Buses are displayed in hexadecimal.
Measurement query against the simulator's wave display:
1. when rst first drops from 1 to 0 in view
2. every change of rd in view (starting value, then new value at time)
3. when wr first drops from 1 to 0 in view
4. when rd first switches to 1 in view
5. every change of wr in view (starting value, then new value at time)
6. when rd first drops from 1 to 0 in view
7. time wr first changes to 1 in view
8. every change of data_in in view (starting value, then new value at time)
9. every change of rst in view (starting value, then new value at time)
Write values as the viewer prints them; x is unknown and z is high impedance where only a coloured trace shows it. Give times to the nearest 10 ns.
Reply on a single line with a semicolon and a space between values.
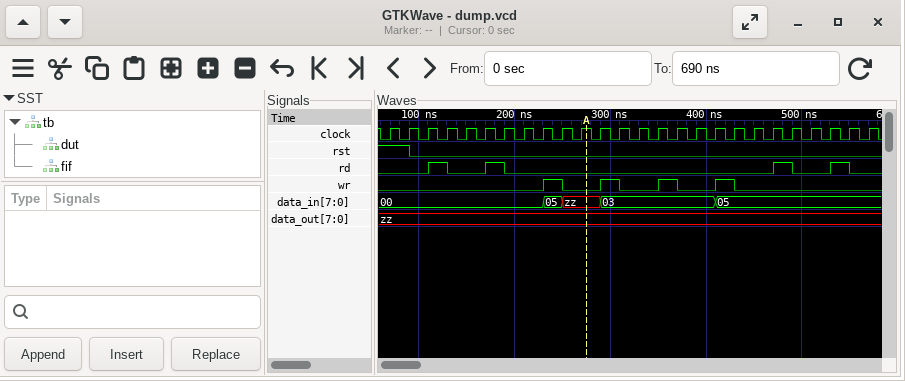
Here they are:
90 ns; 0, 1 at 110 ns, 0 at 130 ns, 1 at 170 ns, 0 at 190 ns, 1 at 470 ns, 0 at 490 ns, 1 at 530 ns, 0 at 550 ns; 250 ns; 110 ns; 0, 1 at 230 ns, 0 at 250 ns, 1 at 290 ns, 0 at 310 ns, 1 at 350 ns, 0 at 370 ns, 1 at 410 ns, 0 at 430 ns; 130 ns; 230 ns; 00, 05 at 230 ns, zz at 250 ns, 03 at 290 ns, 05 at 410 ns; 1, 0 at 90 ns
